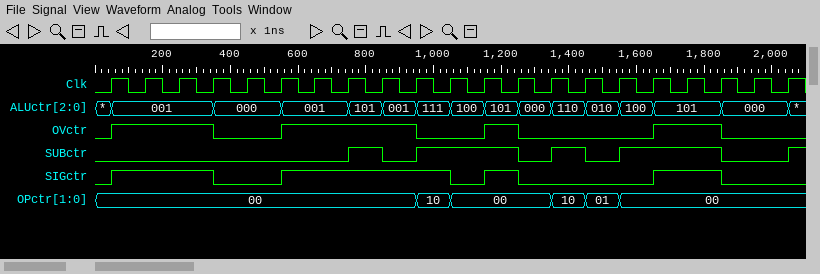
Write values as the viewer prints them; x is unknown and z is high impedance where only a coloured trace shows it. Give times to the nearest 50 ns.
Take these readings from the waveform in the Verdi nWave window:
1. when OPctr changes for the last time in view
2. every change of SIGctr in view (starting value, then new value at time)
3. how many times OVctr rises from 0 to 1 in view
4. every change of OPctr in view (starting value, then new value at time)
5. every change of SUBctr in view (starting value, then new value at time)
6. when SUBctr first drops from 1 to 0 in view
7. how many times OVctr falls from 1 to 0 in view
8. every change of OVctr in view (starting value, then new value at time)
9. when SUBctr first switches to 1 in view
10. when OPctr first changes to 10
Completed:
1550 ns
0, 1 at 50 ns, 0 at 350 ns, 1 at 550 ns, 0 at 1050 ns, 1 at 1150 ns, 0 at 1250 ns, 1 at 1650 ns, 0 at 1850 ns
4
00, 10 at 950 ns, 00 at 1050 ns, 10 at 1350 ns, 01 at 1450 ns, 00 at 1550 ns
0, 1 at 750 ns, 0 at 850 ns, 1 at 950 ns, 0 at 1250 ns, 1 at 1350 ns, 0 at 1450 ns, 1 at 1550 ns, 0 at 1850 ns, 1 at 2050 ns
850 ns
4
0, 1 at 50 ns, 0 at 350 ns, 1 at 550 ns, 0 at 950 ns, 1 at 1150 ns, 0 at 1250 ns, 1 at 1650 ns, 0 at 1850 ns
750 ns
950 ns
